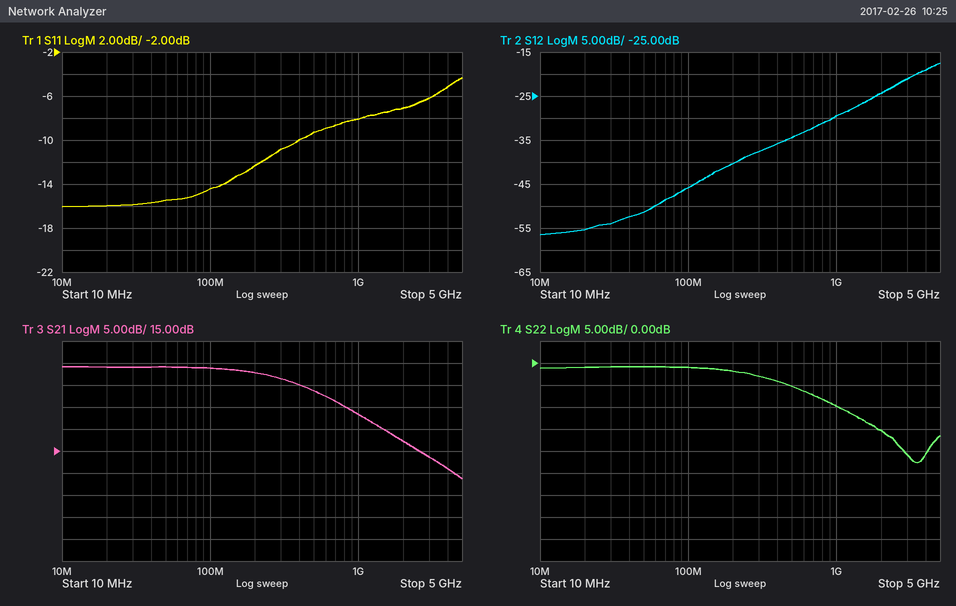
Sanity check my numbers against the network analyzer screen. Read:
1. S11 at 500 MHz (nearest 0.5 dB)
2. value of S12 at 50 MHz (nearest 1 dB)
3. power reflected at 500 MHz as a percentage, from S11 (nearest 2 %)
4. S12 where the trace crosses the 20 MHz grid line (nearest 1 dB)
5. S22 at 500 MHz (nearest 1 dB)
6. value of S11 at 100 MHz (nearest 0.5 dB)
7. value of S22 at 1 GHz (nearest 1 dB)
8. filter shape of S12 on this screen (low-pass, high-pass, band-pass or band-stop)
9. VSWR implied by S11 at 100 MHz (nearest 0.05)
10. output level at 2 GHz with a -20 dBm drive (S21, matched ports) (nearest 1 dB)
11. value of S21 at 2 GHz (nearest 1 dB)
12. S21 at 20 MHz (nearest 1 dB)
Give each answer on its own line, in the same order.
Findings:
-9.5 dB
-51 dB
12 %
-55 dB
-5 dB
-14.5 dB
-10 dB
high-pass
1.45
-3 dBm
17 dB
34 dB
